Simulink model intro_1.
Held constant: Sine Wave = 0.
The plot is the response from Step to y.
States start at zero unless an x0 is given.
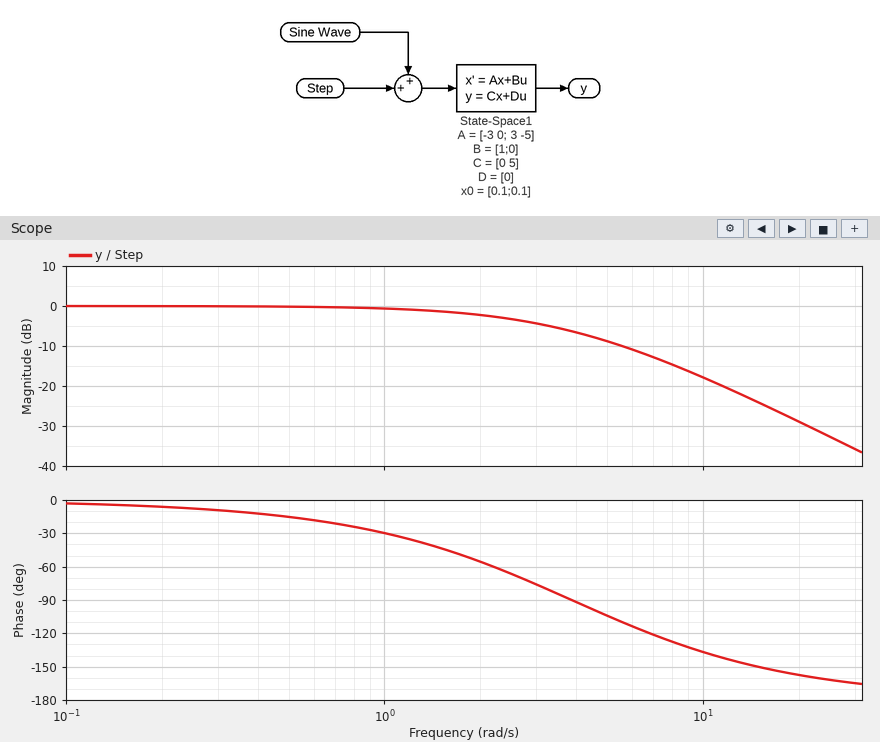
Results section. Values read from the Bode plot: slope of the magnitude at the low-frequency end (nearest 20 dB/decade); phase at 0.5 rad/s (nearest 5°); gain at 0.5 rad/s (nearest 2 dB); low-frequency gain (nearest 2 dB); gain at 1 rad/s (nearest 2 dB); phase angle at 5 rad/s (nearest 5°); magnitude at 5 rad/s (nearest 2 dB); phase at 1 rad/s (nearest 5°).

0 dB/decade
-15°
0 dB
0 dB
0 dB
-105°
-8 dB
-30°
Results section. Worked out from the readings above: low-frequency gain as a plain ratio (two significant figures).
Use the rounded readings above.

1.0
